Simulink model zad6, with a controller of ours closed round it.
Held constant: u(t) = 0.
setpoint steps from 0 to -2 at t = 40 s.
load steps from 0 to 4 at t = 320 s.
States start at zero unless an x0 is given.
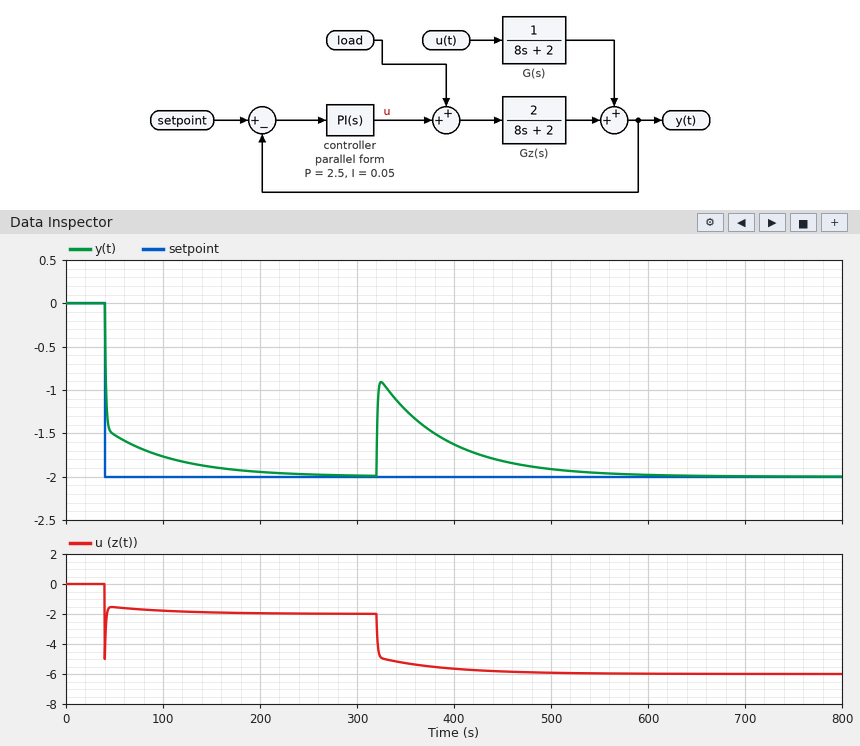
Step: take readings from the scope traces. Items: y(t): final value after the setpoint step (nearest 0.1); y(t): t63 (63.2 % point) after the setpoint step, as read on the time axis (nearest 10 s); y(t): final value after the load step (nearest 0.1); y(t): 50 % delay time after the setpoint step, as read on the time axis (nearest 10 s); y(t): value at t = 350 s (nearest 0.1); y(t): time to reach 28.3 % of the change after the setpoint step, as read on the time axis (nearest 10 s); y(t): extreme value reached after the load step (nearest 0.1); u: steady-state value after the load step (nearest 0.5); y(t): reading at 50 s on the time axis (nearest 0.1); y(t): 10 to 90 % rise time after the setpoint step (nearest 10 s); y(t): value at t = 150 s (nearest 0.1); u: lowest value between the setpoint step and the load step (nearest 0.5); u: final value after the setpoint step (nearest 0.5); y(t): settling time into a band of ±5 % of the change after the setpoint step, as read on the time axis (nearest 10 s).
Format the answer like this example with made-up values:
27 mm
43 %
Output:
-2.0
40 s
-2.0
40 s
-1.2
40 s
-0.9
-6.0
-1.5
70 s
-1.9
-5.0
-2.0
160 s
